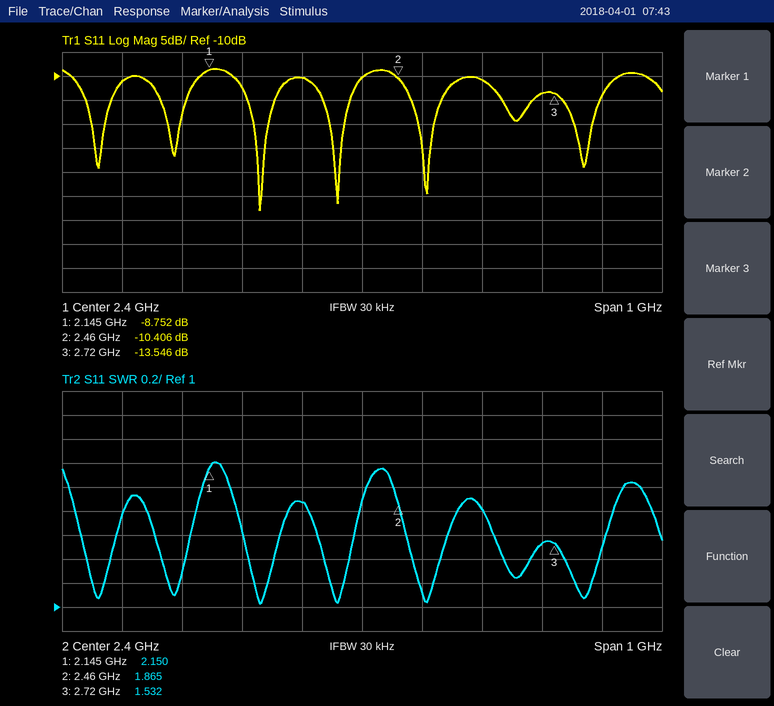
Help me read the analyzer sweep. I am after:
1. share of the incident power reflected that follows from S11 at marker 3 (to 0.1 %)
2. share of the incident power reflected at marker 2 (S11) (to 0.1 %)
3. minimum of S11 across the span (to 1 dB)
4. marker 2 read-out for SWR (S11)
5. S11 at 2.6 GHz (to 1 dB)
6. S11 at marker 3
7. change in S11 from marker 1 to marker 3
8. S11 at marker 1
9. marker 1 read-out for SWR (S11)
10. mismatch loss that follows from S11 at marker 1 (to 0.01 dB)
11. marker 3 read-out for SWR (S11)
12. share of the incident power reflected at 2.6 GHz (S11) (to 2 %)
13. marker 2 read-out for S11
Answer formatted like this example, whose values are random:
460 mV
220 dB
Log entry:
4.4 %
9.1 %
-38 dB
1.865
-11 dB
-13.546 dB
-4.794 dB
-8.752 dB
2.150
0.62 dB
1.532
8 %
-10.406 dB
